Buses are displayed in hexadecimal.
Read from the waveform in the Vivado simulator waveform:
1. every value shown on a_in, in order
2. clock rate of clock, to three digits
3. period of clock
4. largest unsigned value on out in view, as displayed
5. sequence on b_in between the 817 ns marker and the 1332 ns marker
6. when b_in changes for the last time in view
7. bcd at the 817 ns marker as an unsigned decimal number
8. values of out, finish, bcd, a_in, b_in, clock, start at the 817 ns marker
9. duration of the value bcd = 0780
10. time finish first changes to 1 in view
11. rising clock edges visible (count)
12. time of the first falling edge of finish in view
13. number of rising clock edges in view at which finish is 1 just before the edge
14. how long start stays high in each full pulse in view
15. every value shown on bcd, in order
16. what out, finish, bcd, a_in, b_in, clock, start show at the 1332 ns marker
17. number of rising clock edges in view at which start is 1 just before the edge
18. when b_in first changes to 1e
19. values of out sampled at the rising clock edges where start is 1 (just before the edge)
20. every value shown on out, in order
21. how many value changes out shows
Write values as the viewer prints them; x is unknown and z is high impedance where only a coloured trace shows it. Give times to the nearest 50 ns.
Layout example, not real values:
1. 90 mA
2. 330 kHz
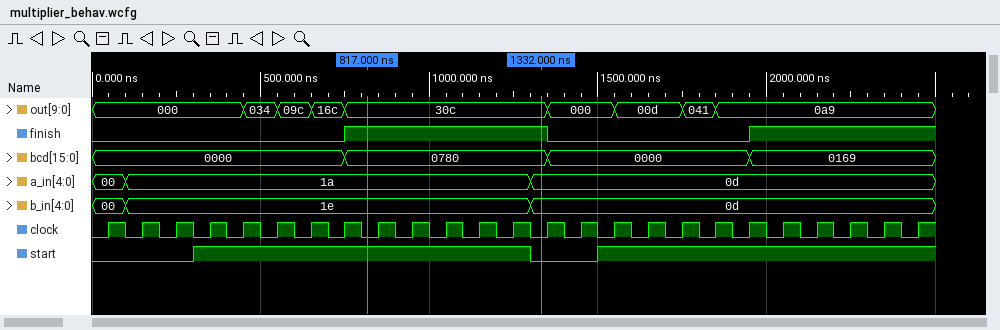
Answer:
1. 00, 1a, 0d
2. 10.0 MHz
3. 100 ns
4. 30c
5. 1e, 0d
6. 1300 ns
7. 1920
8. out=30c, finish=1, bcd=0780, a_in=1a, b_in=1e, clock=0, start=1
9. 600 ns
10. 750 ns
11. 25
12. 1350 ns
13. 11
14. 1000 ns
15. 0000, 0780, 0000, 0169
16. out=30c, finish=1, bcd=0780, a_in=0d, b_in=0d, clock=0, start=0
17. 20
18. 100 ns
19. 000, 000, 034, 09c, 16c, 30c, 30c, 30c, 30c, 30c, 000, 00d, 00d, 041, 0a9, 0a9, 0a9, 0a9, 0a9, 0a9
20. 000, 034, 09c, 16c, 30c, 000, 00d, 041, 0a9
21. 8
